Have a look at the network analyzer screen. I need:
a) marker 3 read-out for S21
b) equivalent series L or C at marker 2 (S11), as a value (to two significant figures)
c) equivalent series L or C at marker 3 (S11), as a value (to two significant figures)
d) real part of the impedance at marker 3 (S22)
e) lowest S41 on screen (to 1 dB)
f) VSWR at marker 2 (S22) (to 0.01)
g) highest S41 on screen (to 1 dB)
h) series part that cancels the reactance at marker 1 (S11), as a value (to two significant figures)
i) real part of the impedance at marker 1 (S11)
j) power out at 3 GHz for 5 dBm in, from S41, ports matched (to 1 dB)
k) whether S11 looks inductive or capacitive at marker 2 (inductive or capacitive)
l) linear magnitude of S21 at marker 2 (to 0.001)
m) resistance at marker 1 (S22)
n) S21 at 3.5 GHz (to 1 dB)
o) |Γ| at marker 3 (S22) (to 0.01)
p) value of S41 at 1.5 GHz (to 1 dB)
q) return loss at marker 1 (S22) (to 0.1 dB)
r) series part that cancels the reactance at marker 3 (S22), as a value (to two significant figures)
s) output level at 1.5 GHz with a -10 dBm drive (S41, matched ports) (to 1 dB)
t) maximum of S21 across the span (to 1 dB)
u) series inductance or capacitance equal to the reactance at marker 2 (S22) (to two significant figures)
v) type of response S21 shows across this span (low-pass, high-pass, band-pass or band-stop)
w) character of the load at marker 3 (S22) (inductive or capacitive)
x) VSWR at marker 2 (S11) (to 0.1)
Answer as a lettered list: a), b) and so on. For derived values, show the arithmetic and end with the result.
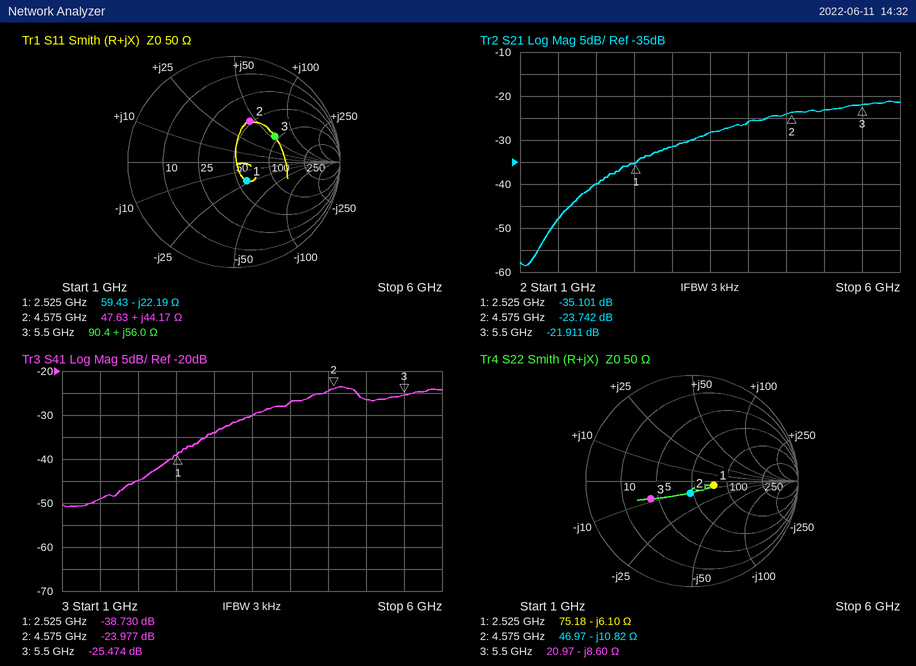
a) -21.911 dB
b) L = 44.17 Ω/(2π × 4.575 GHz) ≈ 1.5 nH
c) L = 56 Ω/(2π × 5.5 GHz) ≈ 1.6 nH
d) 20.97 Ω
e) -51 dB
f) 1.26
g) -24 dB
h) L = 22.19 Ω/(2π × 2.525 GHz) ≈ 1.4 nH
i) 59.43 Ω
j) 5 dBm + (-34 dB) = -29 dBm
k) inductive
l) 10^(-23.742/20) ≈ 0.065
m) 75.18 Ω
n) -28 dB
o) 0.42
p) -49 dB
q) 13.7 dB
r) L = 8.6 Ω/(2π × 5.5 GHz) ≈ 249 pH, so 250 pH to two significant figures
s) -10 dBm + (-49 dB) = -59 dBm
t) -21 dB
u) C = 1/(2π × 4.575 GHz × 10.82 Ω) ≈ 3.2 pF
v) high-pass
w) capacitive
x) 2.4
